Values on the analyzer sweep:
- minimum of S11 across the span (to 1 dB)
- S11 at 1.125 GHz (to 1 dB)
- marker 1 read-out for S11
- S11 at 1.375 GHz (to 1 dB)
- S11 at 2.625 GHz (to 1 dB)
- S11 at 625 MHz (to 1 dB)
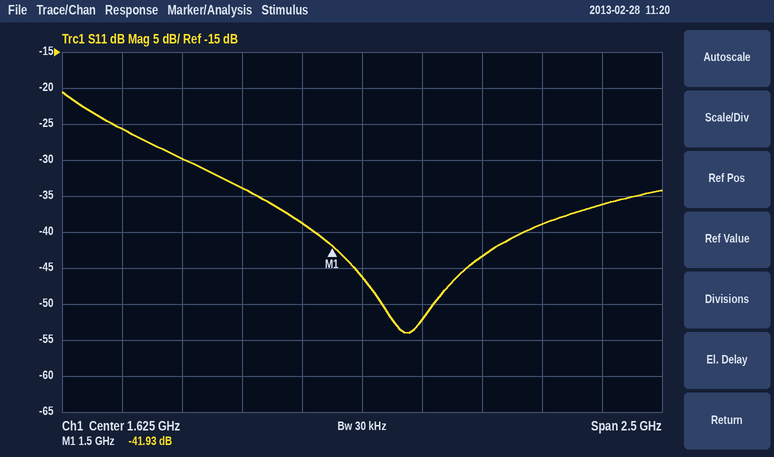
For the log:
-54 dB
-34 dB
-41.93 dB
-39 dB
-36 dB
-26 dB
